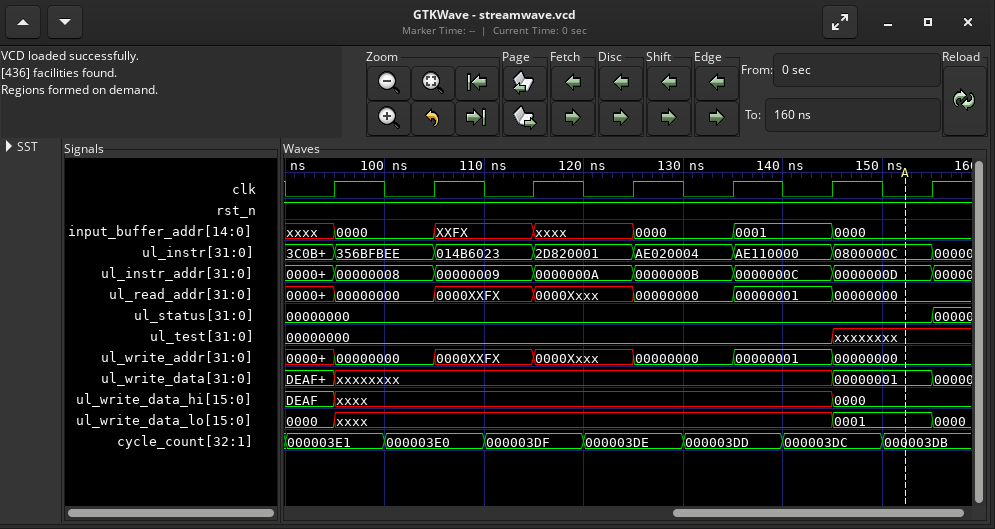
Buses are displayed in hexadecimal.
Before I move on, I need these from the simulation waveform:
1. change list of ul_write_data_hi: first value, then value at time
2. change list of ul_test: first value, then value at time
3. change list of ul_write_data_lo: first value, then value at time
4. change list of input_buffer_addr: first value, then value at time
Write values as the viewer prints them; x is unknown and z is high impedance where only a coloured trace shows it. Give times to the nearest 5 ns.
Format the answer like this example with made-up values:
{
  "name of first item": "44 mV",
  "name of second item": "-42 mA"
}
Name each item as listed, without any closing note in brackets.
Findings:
{
  "change list of ul_write_data_hi: first value, then value at time": "DEAF, xxxx at 95 ns, 0000 at 145 ns",
  "change list of ul_test: first value, then value at time": "00000000, xxxxxxxx at 145 ns",
  "change list of ul_write_data_lo: first value, then value at time": "0000, xxxx at 95 ns, 0001 at 145 ns, 0000 at 155 ns",
  "change list of input_buffer_addr: first value, then value at time": "xxxx, 0000 at 95 ns, XXFX at 105 ns, xxxx at 115 ns, 0000 at 125 ns, 0001 at 135 ns, 0000 at 145 ns"
}
